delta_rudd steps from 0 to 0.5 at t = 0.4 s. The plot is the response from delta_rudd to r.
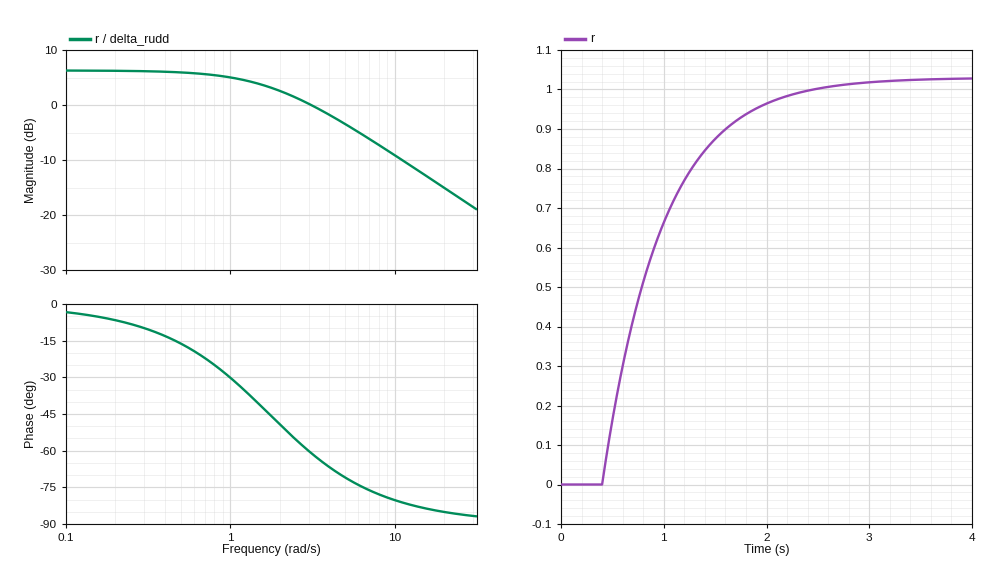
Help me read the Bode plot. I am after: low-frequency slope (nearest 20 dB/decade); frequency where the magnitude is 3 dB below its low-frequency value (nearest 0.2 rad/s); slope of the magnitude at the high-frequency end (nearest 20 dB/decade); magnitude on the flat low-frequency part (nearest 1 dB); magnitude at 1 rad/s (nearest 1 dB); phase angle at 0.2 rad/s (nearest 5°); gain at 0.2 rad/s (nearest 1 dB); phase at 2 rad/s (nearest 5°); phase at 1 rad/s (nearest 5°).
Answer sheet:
0 dB/decade
1.8 rad/s
-20 dB/decade
6 dB
5 dB
-5°
6 dB
-50°
-30°
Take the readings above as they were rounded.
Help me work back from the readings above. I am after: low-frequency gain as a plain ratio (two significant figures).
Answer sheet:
2.0
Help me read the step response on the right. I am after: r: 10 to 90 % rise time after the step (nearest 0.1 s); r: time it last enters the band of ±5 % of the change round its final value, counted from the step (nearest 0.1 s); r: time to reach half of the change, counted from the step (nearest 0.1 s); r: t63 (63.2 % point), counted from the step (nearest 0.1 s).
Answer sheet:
1.3 s
1.7 s
0.4 s
0.6 s
